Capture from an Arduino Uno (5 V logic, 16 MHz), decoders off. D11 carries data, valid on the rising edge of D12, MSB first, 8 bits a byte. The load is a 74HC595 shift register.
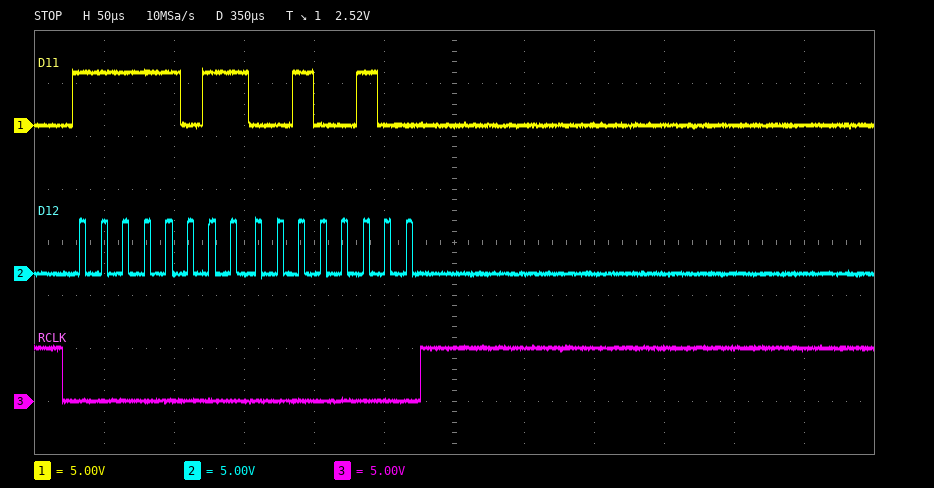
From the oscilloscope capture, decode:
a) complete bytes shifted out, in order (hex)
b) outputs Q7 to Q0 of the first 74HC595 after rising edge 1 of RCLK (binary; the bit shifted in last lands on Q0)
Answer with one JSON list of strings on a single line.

["FB 24", "00100100"]
